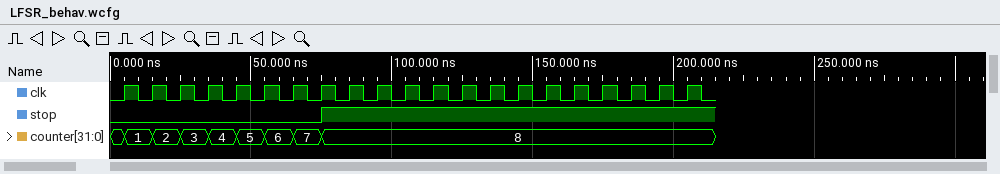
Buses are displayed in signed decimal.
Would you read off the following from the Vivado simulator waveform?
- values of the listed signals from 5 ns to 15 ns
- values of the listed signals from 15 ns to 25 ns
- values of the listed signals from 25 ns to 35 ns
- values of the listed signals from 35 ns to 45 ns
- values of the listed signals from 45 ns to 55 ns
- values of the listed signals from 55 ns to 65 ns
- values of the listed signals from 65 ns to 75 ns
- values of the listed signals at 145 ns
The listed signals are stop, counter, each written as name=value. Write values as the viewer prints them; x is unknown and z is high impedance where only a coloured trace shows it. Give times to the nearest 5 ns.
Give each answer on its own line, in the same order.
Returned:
stop=0, counter=1
stop=0, counter=2
stop=0, counter=3
stop=0, counter=4
stop=0, counter=5
stop=0, counter=6
stop=0, counter=7
stop=1, counter=8
